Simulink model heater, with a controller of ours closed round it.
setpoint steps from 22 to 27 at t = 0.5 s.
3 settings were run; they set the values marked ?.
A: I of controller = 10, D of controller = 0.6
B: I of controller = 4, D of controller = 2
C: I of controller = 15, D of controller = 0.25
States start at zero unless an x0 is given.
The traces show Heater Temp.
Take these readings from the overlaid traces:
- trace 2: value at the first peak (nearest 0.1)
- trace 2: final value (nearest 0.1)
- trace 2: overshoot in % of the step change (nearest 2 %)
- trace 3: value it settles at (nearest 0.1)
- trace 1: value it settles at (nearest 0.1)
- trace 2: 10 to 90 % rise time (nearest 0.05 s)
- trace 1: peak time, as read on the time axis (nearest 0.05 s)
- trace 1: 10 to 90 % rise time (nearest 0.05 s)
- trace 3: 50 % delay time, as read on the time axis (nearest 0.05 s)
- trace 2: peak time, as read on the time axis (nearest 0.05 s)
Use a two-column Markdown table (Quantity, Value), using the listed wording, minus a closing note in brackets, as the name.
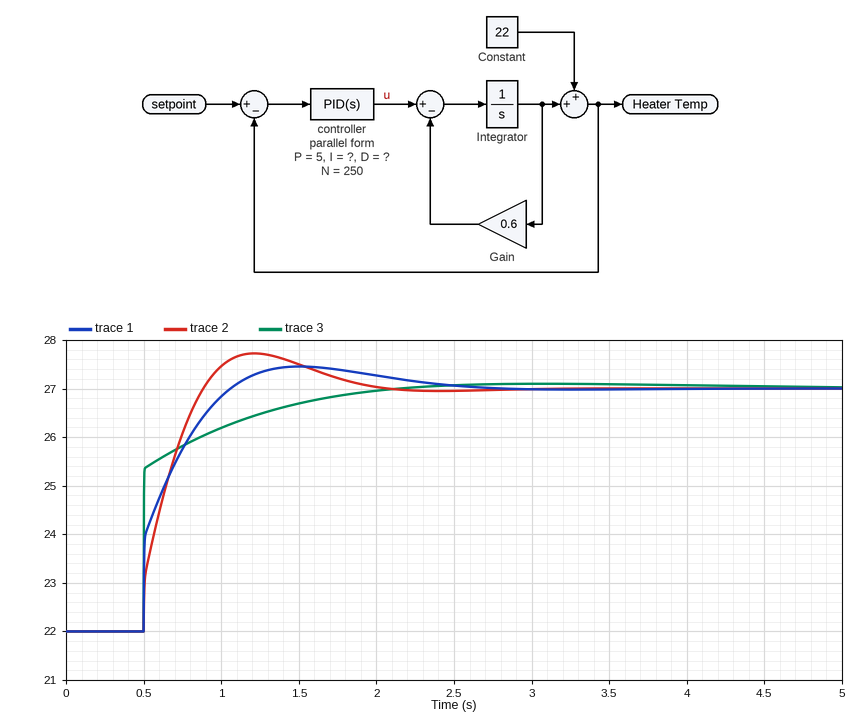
| Quantity | Value |
|---|---|
| trace 2: value at the first peak | 27.7 |
| trace 2: final value | 27.0 |
| trace 2: overshoot in % of the step change | 14 % |
| trace 3: value it settles at | 27.0 |
| trace 1: value it settles at | 27.0 |
| trace 2: 10 to 90 % rise time | 0.30 s |
| trace 1: peak time, as read on the time axis | 1.50 s |
| trace 1: 10 to 90 % rise time | 0.40 s |
| trace 3: 50 % delay time, as read on the time axis | 0.50 s |
| trace 2: peak time, as read on the time axis | 1.20 s |
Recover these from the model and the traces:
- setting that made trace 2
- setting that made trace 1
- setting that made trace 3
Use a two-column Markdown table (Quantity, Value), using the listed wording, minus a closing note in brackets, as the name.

| Quantity | Value |
|---|---|
| setting that made trace 2 | C |
| setting that made trace 1 | A |
| setting that made trace 3 | B |
